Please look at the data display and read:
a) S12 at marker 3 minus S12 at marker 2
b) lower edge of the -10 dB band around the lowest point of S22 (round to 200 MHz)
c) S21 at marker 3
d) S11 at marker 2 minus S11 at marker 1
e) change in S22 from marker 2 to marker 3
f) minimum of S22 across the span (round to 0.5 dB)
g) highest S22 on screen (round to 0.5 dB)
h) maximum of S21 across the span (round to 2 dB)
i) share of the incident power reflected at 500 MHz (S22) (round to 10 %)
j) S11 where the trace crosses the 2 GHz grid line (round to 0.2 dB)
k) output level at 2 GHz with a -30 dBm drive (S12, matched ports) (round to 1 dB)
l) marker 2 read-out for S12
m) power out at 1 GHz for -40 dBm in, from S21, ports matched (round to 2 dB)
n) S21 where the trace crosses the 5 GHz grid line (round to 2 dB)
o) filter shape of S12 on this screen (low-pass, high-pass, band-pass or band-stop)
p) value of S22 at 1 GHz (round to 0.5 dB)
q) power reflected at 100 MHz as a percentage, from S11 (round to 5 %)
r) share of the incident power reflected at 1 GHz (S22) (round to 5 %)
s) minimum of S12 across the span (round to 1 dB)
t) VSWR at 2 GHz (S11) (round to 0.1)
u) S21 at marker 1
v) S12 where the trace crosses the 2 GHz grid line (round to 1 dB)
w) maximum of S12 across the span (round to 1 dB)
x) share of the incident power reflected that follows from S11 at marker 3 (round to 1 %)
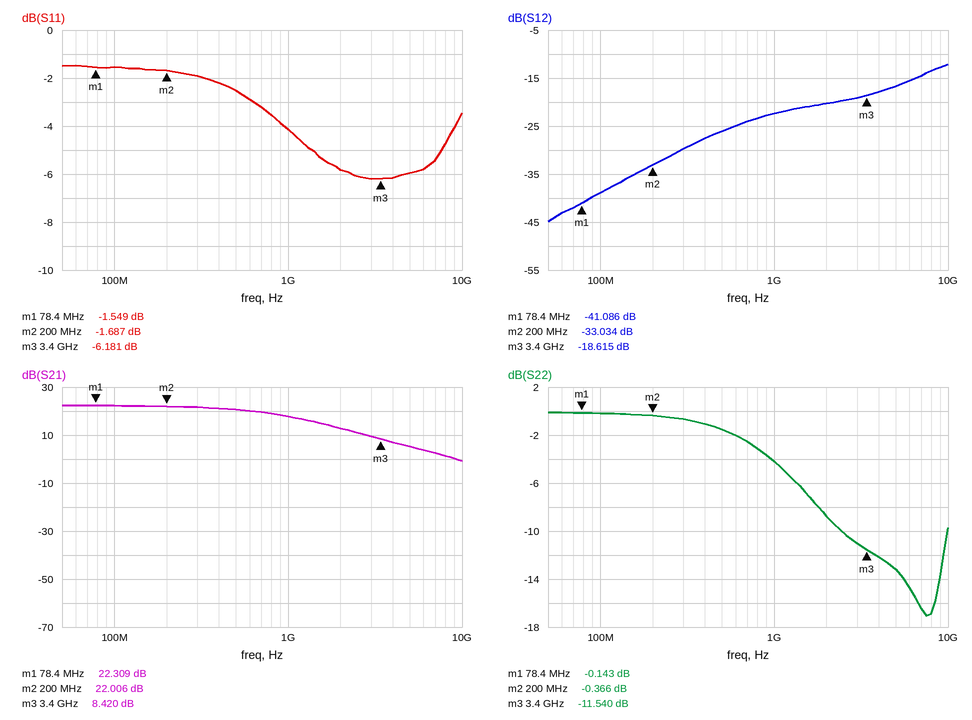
14.419 dB
2.4 GHz
8.420 dB
-0.138 dB
-11.174 dB
-17.0 dB
0.0 dB
22 dB
70 %
-5.8 dB
-50 dBm
-33.034 dB
-22 dBm
6 dB
high-pass
-4.0 dB
70 %
40 %
-45 dB
3.1
22.309 dB
-20 dB
-12 dB
24 %
